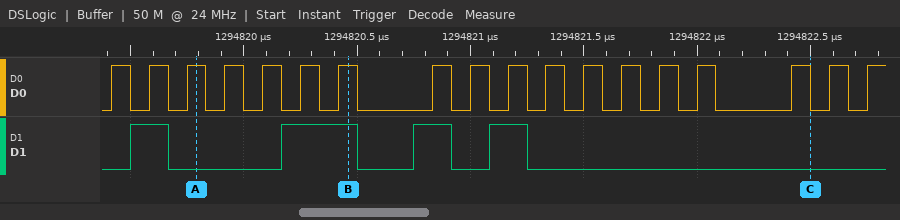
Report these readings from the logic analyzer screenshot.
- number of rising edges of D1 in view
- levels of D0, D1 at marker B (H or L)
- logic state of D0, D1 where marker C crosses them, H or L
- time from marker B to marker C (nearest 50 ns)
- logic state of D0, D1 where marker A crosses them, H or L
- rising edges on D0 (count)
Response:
4
D0=H, D1=H
D0=L, D1=L
2050 ns
D0=H, D1=L
18
